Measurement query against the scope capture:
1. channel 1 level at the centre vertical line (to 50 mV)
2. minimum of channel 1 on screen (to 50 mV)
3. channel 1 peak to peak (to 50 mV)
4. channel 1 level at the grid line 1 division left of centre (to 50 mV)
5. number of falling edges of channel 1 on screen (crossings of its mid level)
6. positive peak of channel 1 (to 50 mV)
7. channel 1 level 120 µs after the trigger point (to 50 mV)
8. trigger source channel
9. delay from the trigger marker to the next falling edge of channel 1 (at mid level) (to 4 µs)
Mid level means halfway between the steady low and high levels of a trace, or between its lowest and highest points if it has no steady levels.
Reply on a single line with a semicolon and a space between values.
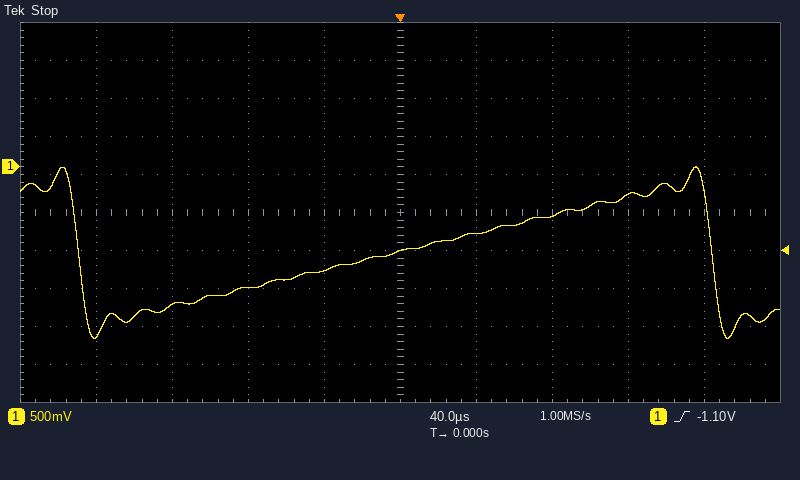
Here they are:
-1.10 V; -2.25 V; 2.25 V; -1.35 V; 2; 0 mV; -350 mV; channel 1; 164 µs
